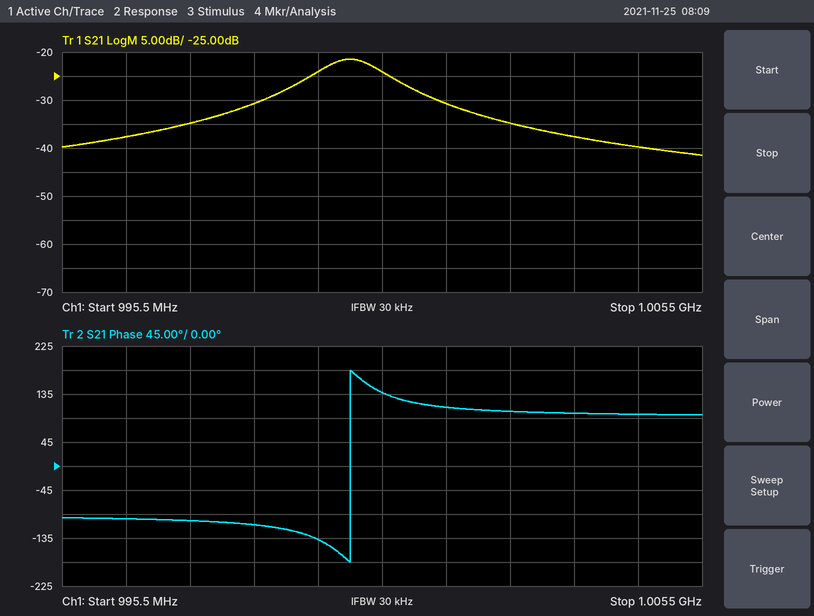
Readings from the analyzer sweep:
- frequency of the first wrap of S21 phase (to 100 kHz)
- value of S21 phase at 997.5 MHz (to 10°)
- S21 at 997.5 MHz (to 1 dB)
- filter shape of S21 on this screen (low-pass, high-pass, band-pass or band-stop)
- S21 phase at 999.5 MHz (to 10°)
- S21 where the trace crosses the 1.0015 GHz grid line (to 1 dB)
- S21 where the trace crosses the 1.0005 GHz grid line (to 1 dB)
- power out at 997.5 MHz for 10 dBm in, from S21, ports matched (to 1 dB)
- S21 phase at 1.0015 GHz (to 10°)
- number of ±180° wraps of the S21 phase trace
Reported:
1.0000 GHz
-100°
-35 dB
band-pass
-140°
-31 dB
-24 dB
-25 dBm
110°
1
